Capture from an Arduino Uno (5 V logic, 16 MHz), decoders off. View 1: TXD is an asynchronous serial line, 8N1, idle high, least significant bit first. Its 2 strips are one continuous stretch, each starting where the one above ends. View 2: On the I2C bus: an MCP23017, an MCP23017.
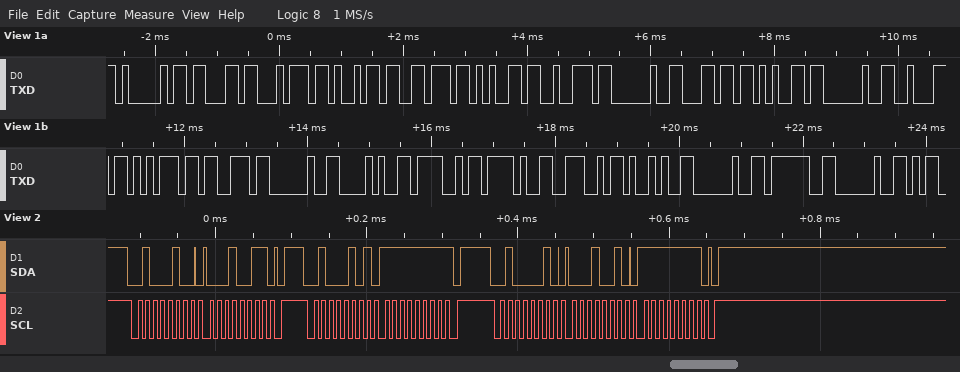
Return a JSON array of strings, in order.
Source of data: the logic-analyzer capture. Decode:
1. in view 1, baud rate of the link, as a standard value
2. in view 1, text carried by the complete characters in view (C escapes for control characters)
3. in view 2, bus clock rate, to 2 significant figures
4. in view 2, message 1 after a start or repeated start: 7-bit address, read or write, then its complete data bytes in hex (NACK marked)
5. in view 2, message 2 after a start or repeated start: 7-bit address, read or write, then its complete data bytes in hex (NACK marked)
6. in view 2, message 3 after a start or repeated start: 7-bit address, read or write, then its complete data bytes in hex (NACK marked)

["9600 baud", "\"Activer le bus (O/N) ? \"", "100 kHz", "0x22 write: 13", "0x22 read: FF NACK", "0x21 write: 12 FF"]
